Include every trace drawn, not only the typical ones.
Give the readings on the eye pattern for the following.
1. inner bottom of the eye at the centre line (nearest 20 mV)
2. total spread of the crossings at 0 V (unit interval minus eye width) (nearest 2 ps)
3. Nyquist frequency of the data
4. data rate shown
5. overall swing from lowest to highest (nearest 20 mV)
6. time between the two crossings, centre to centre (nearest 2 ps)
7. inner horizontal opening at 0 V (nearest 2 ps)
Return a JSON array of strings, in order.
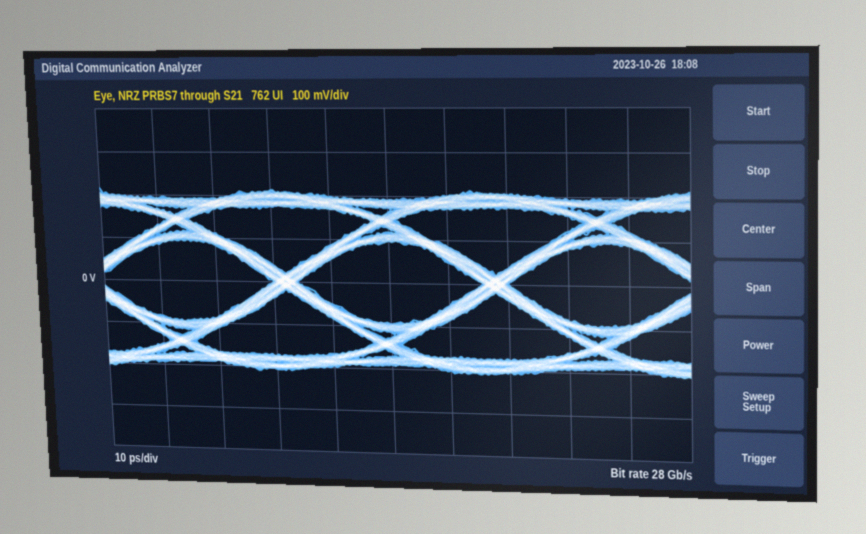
["-100 mV", "4 ps", "14 GHz", "28 Gb/s", "420 mV", "36 ps", "32 ps"]
